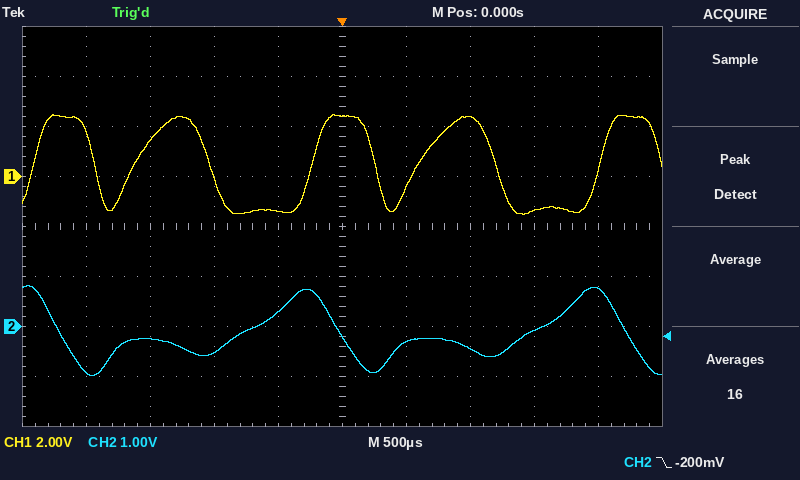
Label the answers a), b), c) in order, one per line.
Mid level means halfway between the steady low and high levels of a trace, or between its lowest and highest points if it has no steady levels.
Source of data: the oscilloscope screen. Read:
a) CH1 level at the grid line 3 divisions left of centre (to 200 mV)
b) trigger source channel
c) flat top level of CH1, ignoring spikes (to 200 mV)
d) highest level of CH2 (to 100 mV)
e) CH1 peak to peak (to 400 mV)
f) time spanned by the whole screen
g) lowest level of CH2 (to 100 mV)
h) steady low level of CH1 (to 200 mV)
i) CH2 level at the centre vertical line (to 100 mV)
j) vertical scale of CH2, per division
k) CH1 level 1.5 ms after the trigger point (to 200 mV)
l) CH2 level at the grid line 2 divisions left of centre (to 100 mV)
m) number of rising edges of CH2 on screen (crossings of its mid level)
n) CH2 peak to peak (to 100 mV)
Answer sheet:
a) 1.4 V
b) CH2
c) 2.4 V
d) 800 mV
e) 4.0 V
f) 5 ms
g) -1.0 V
h) -1.4 V
i) -200 mV
j) 1 V
k) -1.4 V
l) -500 mV
m) 2
n) 1.8 V
